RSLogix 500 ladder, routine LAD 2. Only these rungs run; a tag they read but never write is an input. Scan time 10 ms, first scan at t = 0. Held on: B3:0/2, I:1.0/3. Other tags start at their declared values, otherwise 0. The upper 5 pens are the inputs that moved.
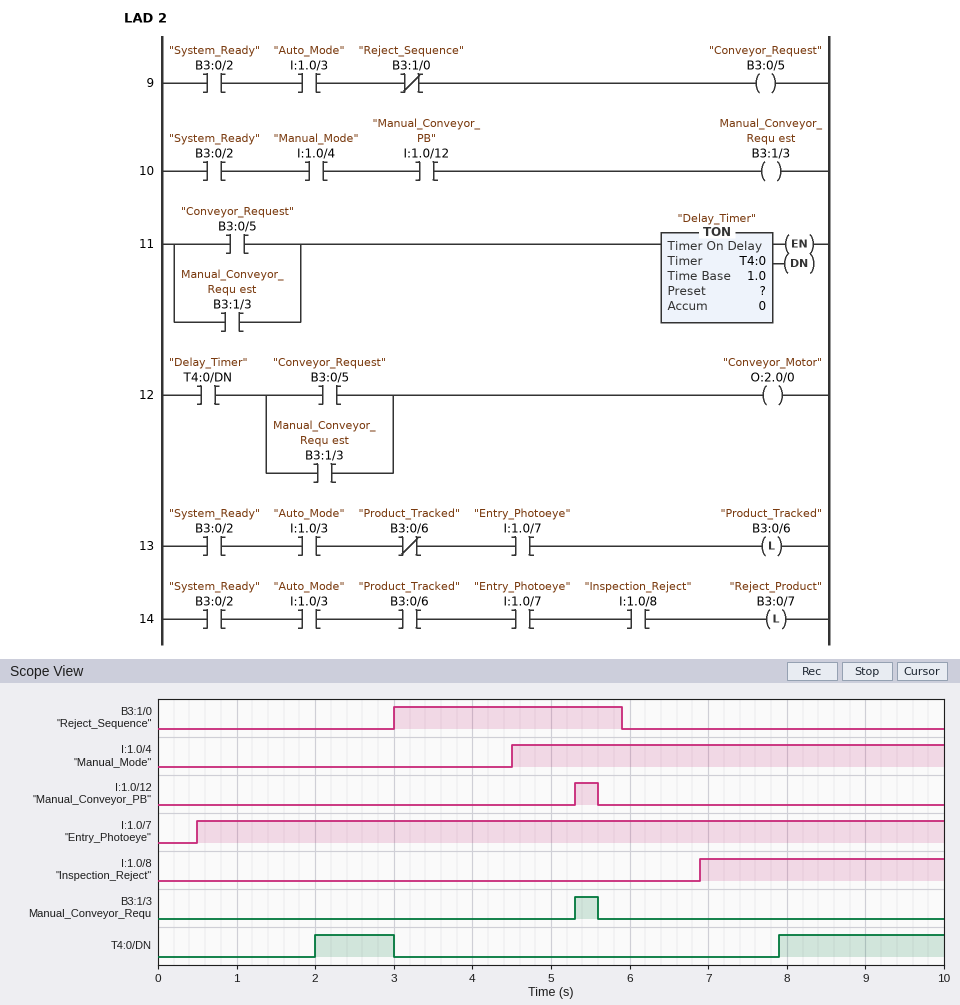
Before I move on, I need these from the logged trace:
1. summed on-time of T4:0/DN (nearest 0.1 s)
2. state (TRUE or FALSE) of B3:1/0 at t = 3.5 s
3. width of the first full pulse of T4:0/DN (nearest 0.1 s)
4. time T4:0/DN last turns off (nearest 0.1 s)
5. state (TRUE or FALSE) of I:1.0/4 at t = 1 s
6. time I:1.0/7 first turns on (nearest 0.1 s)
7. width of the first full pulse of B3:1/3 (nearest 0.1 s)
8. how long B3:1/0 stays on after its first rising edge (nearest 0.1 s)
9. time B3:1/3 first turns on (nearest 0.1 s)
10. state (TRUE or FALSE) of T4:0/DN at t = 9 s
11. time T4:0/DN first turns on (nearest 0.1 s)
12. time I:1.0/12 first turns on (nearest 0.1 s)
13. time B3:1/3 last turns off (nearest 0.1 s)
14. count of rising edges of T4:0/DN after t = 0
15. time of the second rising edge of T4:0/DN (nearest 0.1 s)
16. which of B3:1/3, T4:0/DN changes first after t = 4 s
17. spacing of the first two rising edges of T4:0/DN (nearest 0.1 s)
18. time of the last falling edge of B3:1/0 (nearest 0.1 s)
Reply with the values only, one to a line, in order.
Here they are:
3.1 s
TRUE
1.0 s
3.0 s
FALSE
0.5 s
0.3 s
2.9 s
5.3 s
TRUE
2.0 s
5.3 s
5.6 s
2
7.9 s
B3:1/3
5.9 s
5.9 s
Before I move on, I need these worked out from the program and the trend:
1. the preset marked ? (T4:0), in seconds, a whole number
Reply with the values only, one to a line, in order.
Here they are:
2 s
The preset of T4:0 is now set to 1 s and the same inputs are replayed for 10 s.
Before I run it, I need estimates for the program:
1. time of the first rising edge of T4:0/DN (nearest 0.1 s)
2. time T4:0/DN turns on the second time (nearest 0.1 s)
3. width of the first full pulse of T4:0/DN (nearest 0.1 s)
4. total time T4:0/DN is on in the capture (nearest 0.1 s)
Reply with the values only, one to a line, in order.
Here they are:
1.0 s
6.9 s
2.0 s
5.1 s
